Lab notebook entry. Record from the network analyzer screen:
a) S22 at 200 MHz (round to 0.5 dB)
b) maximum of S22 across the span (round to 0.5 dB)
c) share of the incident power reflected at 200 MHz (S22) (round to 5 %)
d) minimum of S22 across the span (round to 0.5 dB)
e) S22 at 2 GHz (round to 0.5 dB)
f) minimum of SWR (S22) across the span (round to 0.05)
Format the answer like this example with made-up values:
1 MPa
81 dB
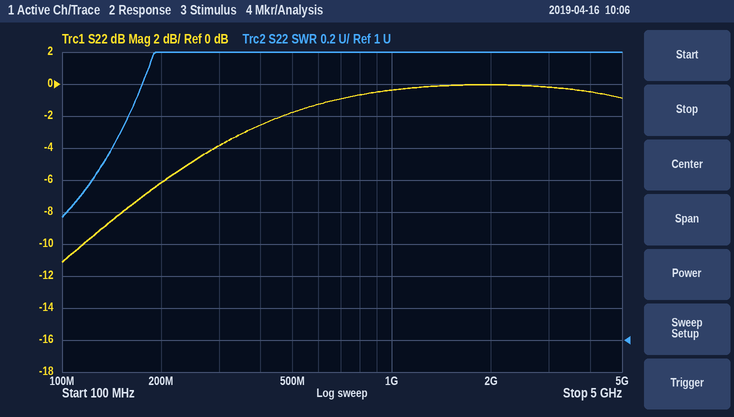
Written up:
-6.0 dB
0.0 dB
25 %
-11.0 dB
0.0 dB
1.75
